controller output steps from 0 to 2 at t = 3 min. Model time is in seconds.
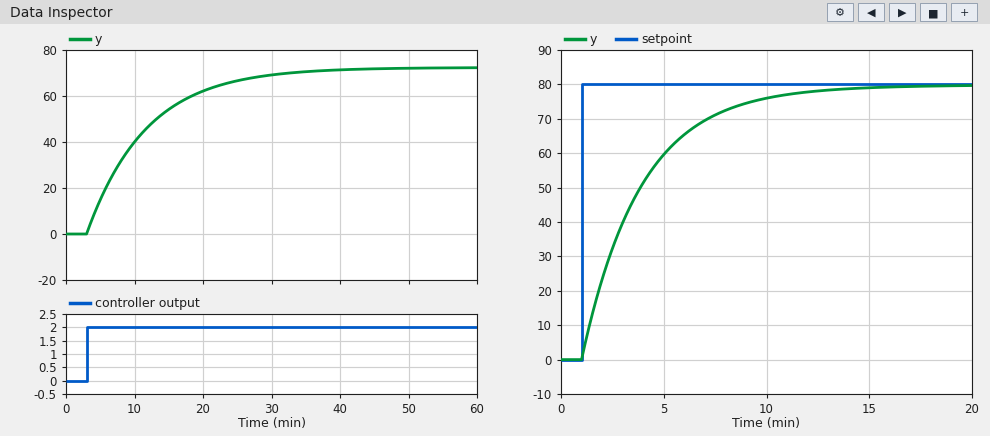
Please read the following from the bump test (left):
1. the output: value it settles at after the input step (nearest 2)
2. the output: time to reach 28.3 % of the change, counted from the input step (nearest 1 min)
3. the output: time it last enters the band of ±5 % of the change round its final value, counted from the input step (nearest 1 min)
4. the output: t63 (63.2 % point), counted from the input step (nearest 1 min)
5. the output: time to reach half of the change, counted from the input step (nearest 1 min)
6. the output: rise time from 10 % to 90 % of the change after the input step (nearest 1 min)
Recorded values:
72
3 min
26 min
9 min
6 min
19 min
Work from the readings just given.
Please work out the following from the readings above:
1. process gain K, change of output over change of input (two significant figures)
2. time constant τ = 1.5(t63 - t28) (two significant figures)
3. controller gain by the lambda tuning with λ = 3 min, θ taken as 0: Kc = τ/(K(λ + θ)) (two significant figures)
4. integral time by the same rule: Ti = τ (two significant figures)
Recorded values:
36
9.0 min
0.083
9.0 min
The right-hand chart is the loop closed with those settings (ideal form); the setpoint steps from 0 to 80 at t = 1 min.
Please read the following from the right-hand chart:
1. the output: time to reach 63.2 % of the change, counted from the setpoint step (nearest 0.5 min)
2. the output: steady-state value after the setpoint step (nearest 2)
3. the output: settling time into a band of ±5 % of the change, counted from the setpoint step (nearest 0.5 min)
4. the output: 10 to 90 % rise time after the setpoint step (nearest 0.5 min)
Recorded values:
3.0 min
80
9.0 min
6.5 min
